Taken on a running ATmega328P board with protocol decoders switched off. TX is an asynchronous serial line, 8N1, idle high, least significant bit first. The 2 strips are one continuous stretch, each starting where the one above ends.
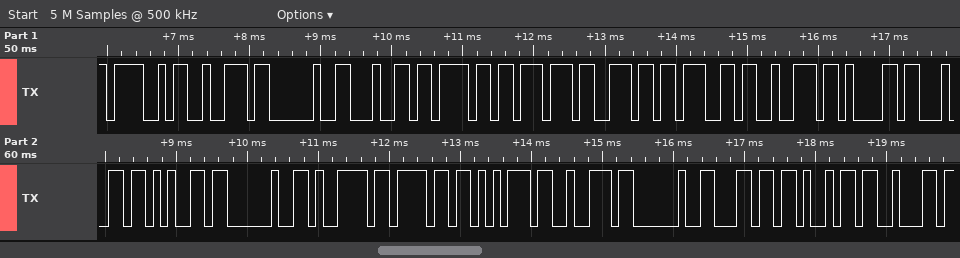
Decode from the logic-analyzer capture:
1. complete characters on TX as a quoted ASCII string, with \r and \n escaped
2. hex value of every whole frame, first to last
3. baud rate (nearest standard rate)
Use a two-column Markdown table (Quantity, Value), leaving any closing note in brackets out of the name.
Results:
| Quantity | Value |
|---|---|
| complete characters on TX as a quoted ASCII string, with \r and \n escaped | "Or downgrade your lib" |
| hex value of every whole frame, first to last | 4F 72 20 64 6F 77 6E 67 72 61 64 65 20 79 6F 75 72 20 6C 69 62 |
| baud rate | 9600 baud |
